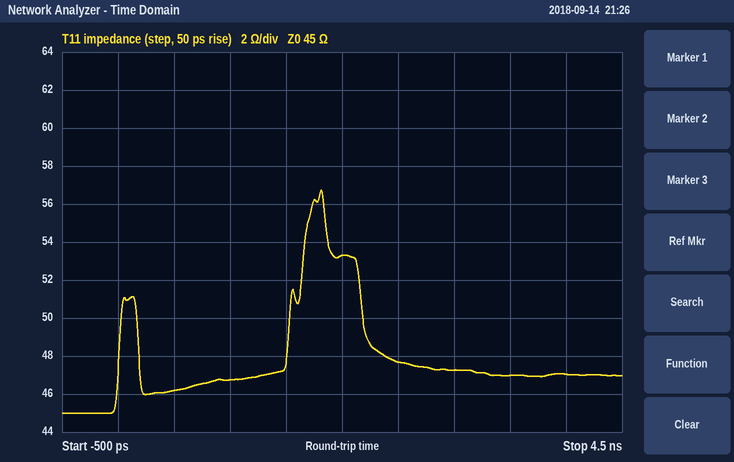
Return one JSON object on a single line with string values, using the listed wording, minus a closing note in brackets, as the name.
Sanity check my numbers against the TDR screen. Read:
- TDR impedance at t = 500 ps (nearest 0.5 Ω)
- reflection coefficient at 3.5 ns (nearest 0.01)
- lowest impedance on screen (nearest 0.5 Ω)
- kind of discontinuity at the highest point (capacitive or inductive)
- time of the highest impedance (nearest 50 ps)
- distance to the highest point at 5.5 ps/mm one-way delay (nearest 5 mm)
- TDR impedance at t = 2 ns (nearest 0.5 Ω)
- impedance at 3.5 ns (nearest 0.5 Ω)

{"TDR impedance at t = 500 ps": "46.0 Ω", "reflection coefficient at 3.5 ns": "+0.02", "lowest impedance on screen": "45.0 Ω", "kind of discontinuity at the highest point": "inductive", "time of the highest impedance": "1.80 ns", "distance to the highest point at 5.5 ps/mm one-way delay": "165 mm", "TDR impedance at t = 2 ns": "53.5 Ω", "impedance at 3.5 ns": "47.0 Ω"}
